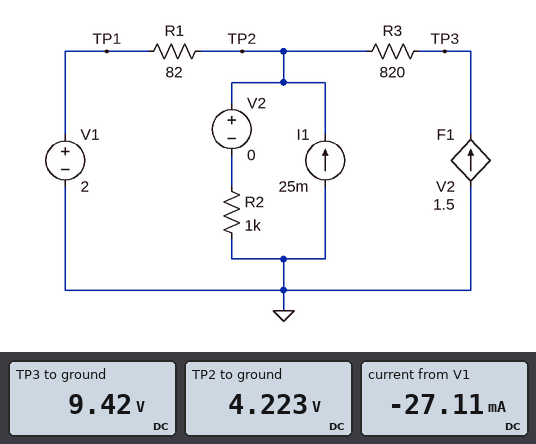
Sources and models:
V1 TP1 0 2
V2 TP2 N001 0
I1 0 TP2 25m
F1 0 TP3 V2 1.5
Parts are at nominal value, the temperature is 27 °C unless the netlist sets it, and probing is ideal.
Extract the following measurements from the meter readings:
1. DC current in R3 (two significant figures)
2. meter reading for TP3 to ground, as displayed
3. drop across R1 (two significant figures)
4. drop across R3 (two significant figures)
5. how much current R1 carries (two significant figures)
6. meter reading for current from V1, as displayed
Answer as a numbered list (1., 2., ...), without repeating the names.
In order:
1. 6.3 mA
2. 9.42 V
3. 2.2 V
4. 5.2 V
5. 27 mA
6. -27.11 mA
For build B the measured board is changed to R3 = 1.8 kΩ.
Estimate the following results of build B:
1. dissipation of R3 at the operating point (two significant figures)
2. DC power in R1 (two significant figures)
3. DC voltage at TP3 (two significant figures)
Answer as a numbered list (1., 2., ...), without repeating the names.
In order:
1. 72 mW
2. 60 mW
3. 16 V
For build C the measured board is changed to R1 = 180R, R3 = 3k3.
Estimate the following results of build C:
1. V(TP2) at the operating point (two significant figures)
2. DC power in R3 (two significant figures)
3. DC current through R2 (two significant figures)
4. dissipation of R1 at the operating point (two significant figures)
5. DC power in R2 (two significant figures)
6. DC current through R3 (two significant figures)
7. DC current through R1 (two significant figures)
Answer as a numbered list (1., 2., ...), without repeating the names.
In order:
1. 7.1 V
2. 380 mW
3. 7.1 mA
4. 150 mW
5. 51 mW
6. 11 mA
7. 29 mA
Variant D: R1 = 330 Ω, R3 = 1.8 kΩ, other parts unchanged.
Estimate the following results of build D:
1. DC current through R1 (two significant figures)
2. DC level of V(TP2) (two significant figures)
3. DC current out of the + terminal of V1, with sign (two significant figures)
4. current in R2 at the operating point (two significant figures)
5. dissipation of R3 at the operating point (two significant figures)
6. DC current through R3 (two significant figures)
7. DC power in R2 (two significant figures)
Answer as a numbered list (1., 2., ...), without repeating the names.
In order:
1. 31 mA
2. 12 V
3. -31 mA
4. 12 mA
5. 610 mW
6. 18 mA
7. 150 mW
